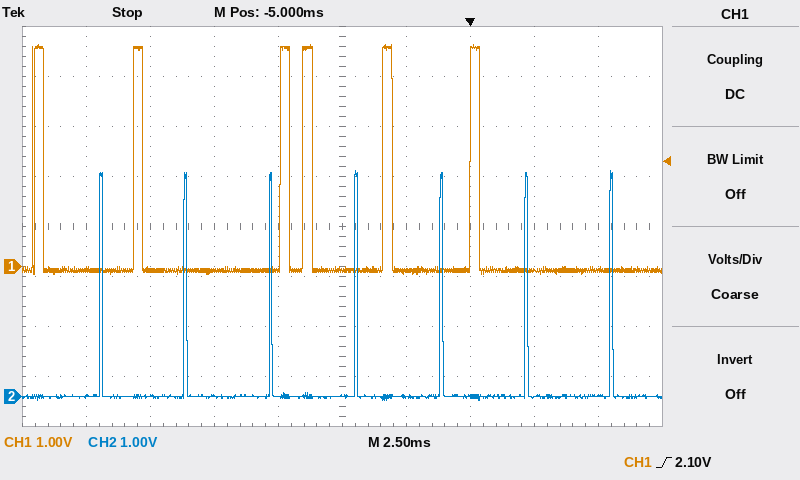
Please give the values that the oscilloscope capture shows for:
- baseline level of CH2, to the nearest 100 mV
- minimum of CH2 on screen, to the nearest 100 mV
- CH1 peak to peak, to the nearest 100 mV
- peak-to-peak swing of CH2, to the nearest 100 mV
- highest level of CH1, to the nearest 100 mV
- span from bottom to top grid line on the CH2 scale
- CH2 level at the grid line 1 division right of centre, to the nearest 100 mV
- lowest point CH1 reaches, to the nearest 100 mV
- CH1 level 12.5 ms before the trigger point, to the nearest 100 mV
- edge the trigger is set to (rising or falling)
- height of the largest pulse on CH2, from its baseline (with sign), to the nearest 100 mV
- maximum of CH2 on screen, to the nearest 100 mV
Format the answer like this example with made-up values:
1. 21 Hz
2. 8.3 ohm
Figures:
1. 0.0 V
2. -100 mV
3. 4.6 V
4. 4.6 V
5. 4.4 V
6. 8 V
7. 0.0 V
8. -200 mV
9. -100 mV
10. rising
11. +4.5 V
12. 4.5 V
